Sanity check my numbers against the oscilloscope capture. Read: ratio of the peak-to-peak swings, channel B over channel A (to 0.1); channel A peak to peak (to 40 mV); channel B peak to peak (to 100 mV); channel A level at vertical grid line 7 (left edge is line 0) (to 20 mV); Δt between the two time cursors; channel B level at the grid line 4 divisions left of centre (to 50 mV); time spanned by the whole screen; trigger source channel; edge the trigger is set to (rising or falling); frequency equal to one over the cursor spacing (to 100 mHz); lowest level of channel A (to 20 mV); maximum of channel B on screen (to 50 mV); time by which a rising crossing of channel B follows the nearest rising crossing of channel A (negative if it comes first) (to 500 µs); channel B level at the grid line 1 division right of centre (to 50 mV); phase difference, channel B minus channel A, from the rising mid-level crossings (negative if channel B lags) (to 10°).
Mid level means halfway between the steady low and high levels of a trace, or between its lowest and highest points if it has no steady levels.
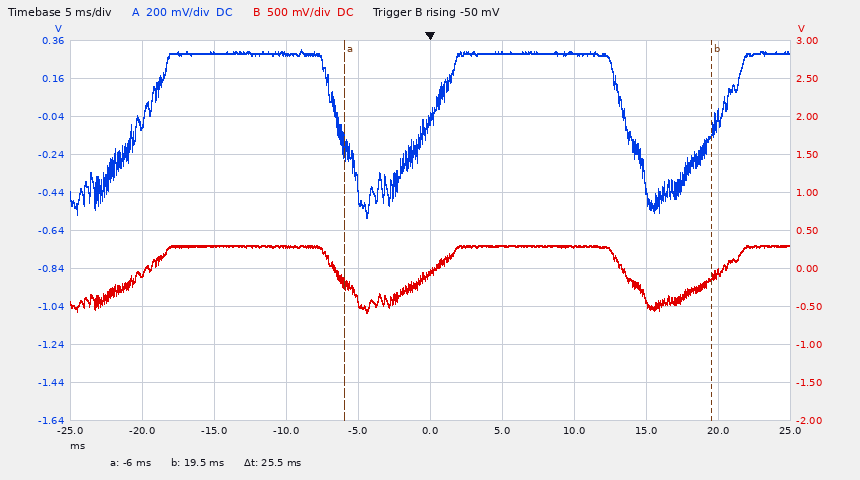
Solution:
1.0
880 mV
900 mV
300 mV
25.5 ms
-50 mV
50 ms
channel B
rising
39.2 Hz
-580 mV
300 mV
0.0 ms
300 mV
0°
